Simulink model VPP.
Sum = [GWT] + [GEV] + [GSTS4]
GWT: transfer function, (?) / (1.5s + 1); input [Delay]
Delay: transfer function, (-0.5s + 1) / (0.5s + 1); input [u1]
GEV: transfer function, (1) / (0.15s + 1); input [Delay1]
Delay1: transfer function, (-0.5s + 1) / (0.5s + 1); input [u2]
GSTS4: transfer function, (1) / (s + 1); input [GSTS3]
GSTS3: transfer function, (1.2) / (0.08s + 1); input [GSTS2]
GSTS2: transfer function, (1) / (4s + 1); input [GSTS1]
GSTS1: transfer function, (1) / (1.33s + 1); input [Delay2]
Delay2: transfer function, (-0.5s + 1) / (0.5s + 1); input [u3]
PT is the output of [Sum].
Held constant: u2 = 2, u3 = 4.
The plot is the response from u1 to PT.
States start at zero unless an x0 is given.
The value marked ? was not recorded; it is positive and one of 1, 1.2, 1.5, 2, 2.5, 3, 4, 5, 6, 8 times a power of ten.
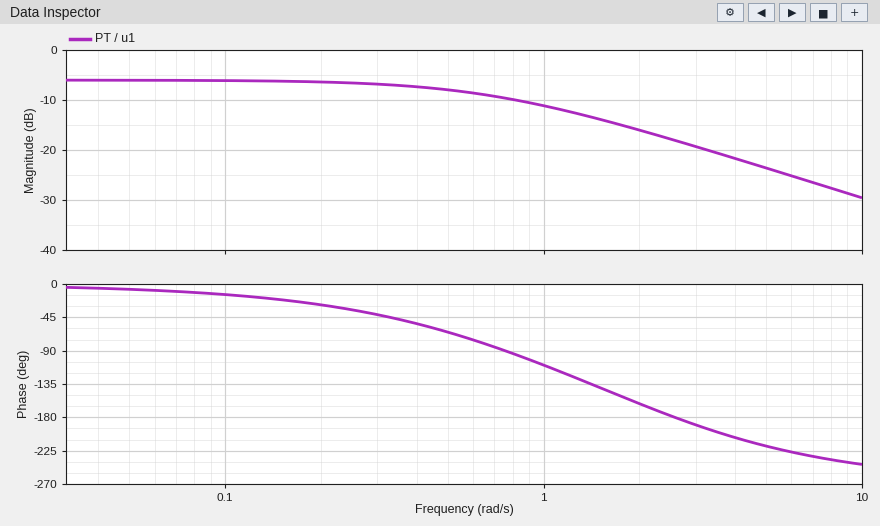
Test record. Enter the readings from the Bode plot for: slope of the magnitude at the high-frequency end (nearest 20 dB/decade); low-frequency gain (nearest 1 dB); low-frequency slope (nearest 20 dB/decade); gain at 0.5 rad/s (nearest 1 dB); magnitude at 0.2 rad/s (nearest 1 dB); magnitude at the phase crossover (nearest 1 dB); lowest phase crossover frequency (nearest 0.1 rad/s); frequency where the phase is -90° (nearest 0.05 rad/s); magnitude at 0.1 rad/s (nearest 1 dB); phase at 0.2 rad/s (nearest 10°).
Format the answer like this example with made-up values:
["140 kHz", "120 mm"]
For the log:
["-20 dB/decade", "-6 dB", "0 dB/decade", "-8 dB", "-6 dB", "-18 dB", "2.6 rad/s", "0.75 rad/s", "-6 dB", "-30°"]
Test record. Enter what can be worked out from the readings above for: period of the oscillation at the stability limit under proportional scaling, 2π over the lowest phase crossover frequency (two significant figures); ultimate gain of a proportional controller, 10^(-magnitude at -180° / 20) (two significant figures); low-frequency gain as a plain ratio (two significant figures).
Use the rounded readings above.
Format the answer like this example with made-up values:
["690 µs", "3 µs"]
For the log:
["2.4 s", "7.9", "0.50"]
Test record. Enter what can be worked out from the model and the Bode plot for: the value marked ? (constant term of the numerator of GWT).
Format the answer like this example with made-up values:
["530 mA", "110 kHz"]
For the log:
["0.5"]
